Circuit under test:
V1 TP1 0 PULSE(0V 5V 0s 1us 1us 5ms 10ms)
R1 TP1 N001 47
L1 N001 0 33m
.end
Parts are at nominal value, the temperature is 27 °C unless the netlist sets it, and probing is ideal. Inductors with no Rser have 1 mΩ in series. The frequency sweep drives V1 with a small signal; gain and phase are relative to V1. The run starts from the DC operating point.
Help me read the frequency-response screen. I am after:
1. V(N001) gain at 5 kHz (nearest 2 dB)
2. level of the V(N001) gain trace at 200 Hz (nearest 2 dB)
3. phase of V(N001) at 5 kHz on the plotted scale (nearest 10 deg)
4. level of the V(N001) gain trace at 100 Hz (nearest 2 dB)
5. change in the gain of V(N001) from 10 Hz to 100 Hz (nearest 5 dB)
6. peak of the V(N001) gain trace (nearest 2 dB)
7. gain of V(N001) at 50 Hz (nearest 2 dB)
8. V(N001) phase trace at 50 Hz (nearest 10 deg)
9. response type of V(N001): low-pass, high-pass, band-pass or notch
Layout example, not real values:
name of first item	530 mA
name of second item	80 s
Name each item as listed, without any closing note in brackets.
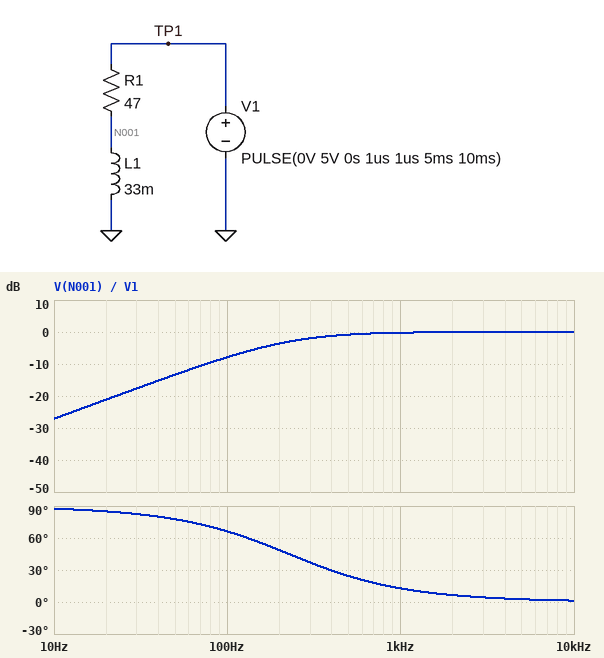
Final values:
V(N001) gain at 5 kHz	0 dB
level of the V(N001) gain trace at 200 Hz	-4 dB
phase of V(N001) at 5 kHz on the plotted scale	0 deg
level of the V(N001) gain trace at 100 Hz	-8 dB
change in the gain of V(N001) from 10 Hz to 100 Hz	20 dB
peak of the V(N001) gain trace	0 dB
gain of V(N001) at 50 Hz	-14 dB
V(N001) phase trace at 50 Hz	80 deg
response type of V(N001): low-pass, high-pass, band-pass or notch	high-pass
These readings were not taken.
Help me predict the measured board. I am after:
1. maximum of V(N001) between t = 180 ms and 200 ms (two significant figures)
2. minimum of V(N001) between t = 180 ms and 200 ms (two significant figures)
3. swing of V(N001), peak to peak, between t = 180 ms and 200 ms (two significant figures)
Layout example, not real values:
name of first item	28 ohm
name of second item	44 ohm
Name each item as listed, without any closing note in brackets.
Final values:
maximum of V(N001) between t = 180 ms and 200 ms	5.0 V
minimum of V(N001) between t = 180 ms and 200 ms	-5.0 V
swing of V(N001), peak to peak, between t = 180 ms and 200 ms	10 V
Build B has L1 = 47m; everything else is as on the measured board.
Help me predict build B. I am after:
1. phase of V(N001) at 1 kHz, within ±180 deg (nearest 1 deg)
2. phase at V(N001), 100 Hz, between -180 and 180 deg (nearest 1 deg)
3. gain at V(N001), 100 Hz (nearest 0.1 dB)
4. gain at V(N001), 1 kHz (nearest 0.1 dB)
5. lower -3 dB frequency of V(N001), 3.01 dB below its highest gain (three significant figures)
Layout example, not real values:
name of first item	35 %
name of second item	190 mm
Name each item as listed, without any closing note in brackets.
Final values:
phase of V(N001) at 1 kHz, within ±180 deg	9 deg
phase at V(N001), 100 Hz, between -180 and 180 deg	58 deg
gain at V(N001), 100 Hz	-5.5 dB
gain at V(N001), 1 kHz	-0.1 dB
lower -3 dB frequency of V(N001), 3.01 dB below its highest gain	159 Hz
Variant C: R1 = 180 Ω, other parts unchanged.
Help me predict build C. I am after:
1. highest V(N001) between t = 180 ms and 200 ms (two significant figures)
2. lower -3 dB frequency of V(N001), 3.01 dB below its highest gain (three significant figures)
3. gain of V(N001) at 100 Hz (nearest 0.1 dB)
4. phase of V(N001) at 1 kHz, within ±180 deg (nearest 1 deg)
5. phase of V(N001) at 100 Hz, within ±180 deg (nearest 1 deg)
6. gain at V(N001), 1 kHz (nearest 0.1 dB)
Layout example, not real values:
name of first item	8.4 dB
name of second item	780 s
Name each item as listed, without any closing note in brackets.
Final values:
highest V(N001) between t = 180 ms and 200 ms	5.0 V
lower -3 dB frequency of V(N001), 3.01 dB below its highest gain	868 Hz
gain of V(N001) at 100 Hz	-18.8 dB
phase of V(N001) at 1 kHz, within ±180 deg	41 deg
phase of V(N001) at 100 Hz, within ±180 deg	83 deg
gain at V(N001), 1 kHz	-2.4 dB
